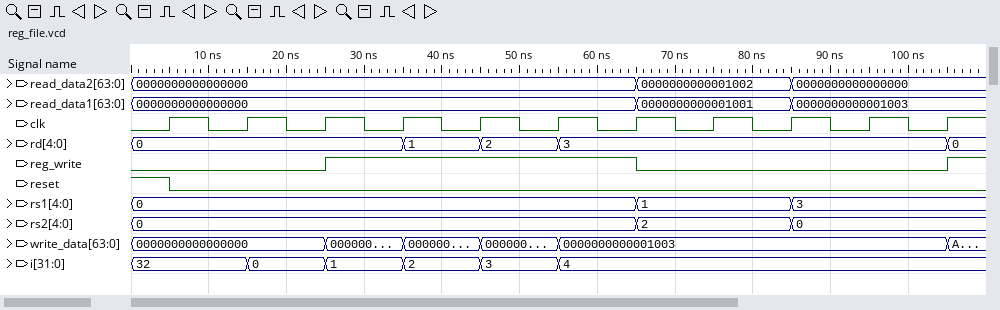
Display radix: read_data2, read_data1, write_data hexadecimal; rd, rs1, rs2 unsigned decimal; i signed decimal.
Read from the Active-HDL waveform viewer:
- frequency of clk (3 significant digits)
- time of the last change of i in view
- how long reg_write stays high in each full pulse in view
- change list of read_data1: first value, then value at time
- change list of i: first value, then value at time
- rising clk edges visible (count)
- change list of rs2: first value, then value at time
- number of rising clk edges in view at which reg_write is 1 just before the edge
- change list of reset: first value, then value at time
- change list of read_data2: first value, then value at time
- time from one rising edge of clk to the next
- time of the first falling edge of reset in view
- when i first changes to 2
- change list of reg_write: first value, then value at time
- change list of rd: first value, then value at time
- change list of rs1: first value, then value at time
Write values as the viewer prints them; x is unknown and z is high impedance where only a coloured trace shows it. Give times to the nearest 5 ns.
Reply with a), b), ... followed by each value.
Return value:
a) 100 MHz
b) 55 ns
c) 40 ns
d) 0000000000000000, 0000000000001001 at 65 ns, 0000000000001003 at 85 ns
e) 32, 0 at 15 ns, 1 at 25 ns, 2 at 35 ns, 3 at 45 ns, 4 at 55 ns
f) 11
g) 0, 2 at 65 ns, 0 at 85 ns
h) 4
i) 1, 0 at 5 ns
j) 0000000000000000, 0000000000001002 at 65 ns, 0000000000000000 at 85 ns
k) 10 ns
l) 5 ns
m) 35 ns
n) 0, 1 at 25 ns, 0 at 65 ns, 1 at 105 ns
o) 0, 1 at 35 ns, 2 at 45 ns, 3 at 55 ns, 0 at 105 ns
p) 0, 1 at 65 ns, 3 at 85 ns
